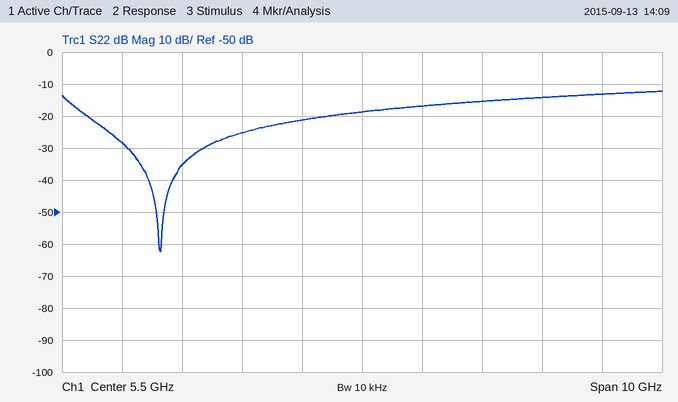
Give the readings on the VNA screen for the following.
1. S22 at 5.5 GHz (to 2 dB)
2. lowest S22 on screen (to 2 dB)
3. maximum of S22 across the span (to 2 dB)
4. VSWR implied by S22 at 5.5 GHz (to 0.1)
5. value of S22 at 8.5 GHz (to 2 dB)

-18 dB
-62 dB
-12 dB
1.3
-14 dB
